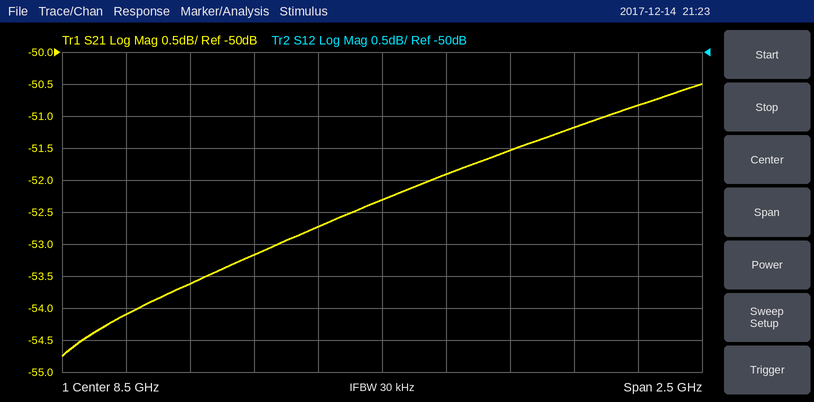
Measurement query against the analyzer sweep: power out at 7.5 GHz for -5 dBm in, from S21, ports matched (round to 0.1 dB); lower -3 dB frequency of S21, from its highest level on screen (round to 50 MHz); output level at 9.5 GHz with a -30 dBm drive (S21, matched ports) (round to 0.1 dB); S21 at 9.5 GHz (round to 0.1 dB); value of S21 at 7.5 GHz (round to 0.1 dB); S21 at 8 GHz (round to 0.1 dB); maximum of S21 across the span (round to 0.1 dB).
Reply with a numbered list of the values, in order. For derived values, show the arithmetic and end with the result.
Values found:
1. -5 dBm + (-54.1 dB) = -59.1 dBm
2. 7.80 GHz
3. -30 dBm + (-50.8 dB) = -80.8 dBm
4. -50.8 dB
5. -54.1 dB
6. -53.2 dB
7. -50.5 dB
